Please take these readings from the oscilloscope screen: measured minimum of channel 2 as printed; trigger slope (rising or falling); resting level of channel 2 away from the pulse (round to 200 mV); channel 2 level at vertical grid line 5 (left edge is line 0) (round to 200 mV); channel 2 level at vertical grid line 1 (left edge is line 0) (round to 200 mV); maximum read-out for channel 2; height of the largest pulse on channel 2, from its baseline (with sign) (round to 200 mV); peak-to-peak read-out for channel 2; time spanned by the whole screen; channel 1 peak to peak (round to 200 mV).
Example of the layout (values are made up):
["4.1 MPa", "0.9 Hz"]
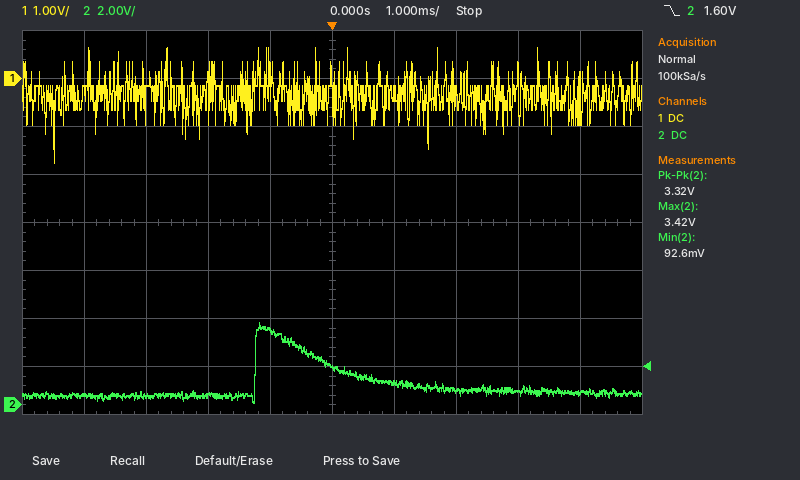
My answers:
["92.6 mV", "falling", "400 mV", "1.6 V", "400 mV", "3.42 V", "+3.0 V", "3.32 V", "10 ms", "2.4 V"]
